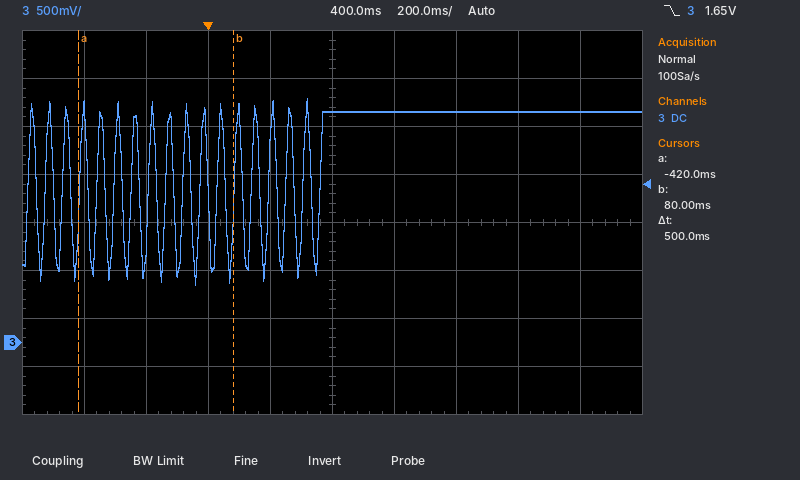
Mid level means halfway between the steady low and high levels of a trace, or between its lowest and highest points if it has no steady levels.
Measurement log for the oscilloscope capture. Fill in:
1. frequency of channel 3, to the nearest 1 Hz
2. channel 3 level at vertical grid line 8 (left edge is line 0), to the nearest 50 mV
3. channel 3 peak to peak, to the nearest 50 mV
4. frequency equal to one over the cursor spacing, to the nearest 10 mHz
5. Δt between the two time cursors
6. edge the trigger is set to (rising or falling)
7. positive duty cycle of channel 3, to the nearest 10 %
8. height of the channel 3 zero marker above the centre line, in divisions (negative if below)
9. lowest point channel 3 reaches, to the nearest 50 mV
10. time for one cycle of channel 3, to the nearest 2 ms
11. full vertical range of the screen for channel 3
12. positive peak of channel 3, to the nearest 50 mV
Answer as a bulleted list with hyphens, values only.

- 18 Hz
- 2.40 V
- 1.95 V
- 2.00 Hz
- 500 ms
- falling
- 50 %
- -2.5 div
- 600 mV
- 56 ms
- 4 V
- 2.55 V
